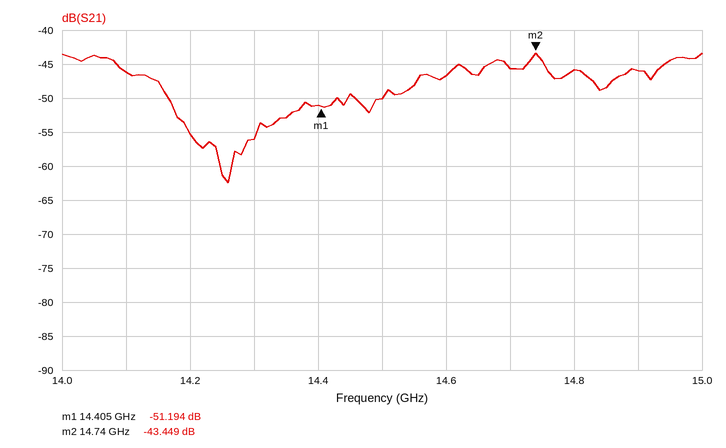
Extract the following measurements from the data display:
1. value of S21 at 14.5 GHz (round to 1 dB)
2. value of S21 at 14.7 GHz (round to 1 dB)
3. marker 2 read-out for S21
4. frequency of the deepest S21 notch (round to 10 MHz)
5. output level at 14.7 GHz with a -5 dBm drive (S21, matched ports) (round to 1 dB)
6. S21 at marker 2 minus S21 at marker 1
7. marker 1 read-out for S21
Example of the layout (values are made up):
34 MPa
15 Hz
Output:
-50 dB
-46 dB
-43.449 dB
14.26 GHz
-51 dBm
7.745 dB
-51.194 dB
